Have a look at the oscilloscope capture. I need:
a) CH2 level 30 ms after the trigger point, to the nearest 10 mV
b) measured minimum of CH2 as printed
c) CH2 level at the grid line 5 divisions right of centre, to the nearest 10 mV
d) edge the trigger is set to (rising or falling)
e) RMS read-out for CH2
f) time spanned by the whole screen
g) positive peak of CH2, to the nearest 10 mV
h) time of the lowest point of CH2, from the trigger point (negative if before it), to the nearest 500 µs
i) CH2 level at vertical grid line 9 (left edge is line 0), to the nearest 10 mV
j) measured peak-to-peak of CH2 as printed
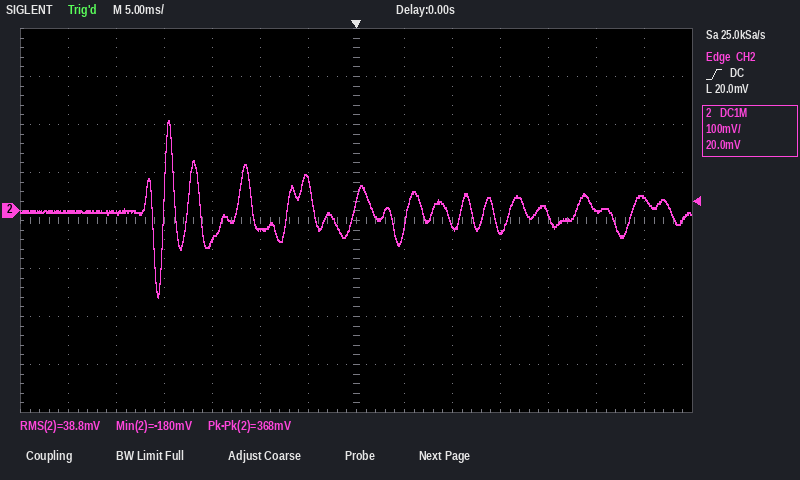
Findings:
30 mV
-180 mV
0 mV
rising
38.8 mV
70 ms
190 mV
-20.5 ms
-30 mV
368 mV
